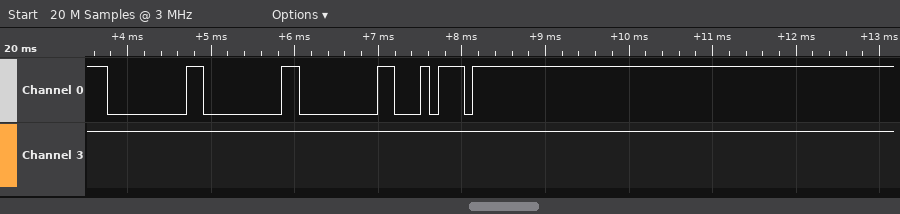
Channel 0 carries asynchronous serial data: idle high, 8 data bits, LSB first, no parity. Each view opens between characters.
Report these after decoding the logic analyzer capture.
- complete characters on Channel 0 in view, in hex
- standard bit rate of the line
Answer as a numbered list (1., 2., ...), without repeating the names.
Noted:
1. 00, 00, 00, 74
2. 9600 baud
